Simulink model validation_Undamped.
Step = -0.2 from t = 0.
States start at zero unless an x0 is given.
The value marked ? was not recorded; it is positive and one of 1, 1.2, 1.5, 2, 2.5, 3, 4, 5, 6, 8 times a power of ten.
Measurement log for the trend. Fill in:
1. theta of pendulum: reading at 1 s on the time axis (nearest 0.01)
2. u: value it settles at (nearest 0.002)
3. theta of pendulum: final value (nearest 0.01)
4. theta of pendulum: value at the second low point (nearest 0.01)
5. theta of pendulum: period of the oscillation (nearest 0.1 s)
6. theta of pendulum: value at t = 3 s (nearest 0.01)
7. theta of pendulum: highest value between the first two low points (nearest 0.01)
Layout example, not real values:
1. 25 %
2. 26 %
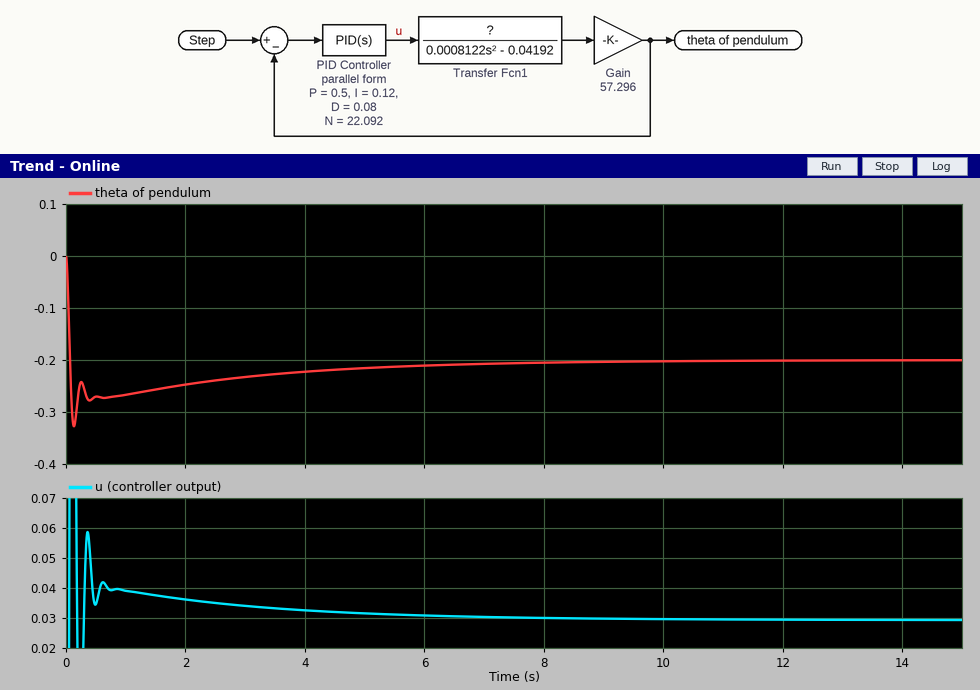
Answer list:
1. -0.27
2. 0.030
3. -0.20
4. -0.28
5. 0.3 s
6. -0.23
7. -0.24
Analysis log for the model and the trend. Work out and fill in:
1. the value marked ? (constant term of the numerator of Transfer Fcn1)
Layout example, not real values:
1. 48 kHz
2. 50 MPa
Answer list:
1. 0.005
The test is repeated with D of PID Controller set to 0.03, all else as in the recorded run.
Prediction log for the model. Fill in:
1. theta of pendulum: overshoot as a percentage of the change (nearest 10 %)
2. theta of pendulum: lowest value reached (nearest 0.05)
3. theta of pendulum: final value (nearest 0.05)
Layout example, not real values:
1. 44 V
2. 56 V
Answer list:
1. 100 %
2. -0.40
3. -0.20
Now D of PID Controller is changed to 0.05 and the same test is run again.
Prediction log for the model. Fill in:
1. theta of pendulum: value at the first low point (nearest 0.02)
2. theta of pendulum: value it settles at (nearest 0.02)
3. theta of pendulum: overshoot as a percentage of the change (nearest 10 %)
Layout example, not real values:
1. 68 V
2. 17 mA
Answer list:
1. -0.36
2. -0.20
3. 80 %
